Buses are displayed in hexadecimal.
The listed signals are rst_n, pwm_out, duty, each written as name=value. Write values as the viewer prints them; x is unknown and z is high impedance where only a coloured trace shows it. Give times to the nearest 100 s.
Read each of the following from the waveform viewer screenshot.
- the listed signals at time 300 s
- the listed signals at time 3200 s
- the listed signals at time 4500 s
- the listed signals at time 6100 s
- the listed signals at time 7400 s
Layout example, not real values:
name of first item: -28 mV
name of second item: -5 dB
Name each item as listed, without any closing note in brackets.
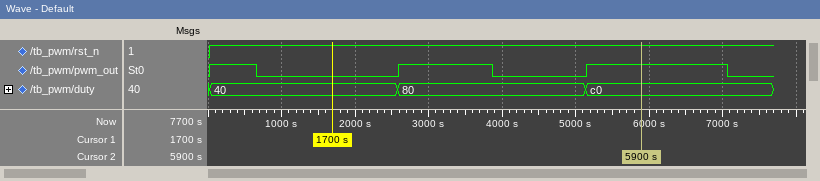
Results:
the listed signals at time 300 s: rst_n=1, pwm_out=1, duty=40
the listed signals at time 3200 s: rst_n=1, pwm_out=1, duty=80
the listed signals at time 4500 s: rst_n=1, pwm_out=0, duty=80
the listed signals at time 6100 s: rst_n=1, pwm_out=1, duty=c0
the listed signals at time 7400 s: rst_n=1, pwm_out=0, duty=c0
